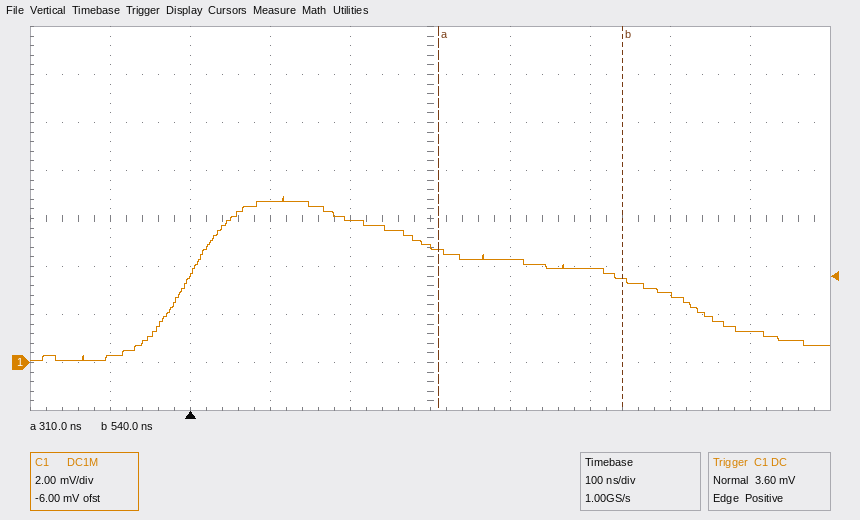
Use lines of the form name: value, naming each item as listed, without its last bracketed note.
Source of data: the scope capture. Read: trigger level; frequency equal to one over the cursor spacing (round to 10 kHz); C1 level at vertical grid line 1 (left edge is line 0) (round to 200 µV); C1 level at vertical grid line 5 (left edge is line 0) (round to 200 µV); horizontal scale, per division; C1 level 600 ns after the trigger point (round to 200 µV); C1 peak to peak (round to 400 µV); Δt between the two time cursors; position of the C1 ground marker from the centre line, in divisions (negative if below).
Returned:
trigger level: 3.60 mV
frequency equal to one over the cursor spacing: 4.35 MHz
C1 level at vertical grid line 1 (left edge is line 0): 200 µV
C1 level at vertical grid line 5 (left edge is line 0): 4.8 mV
horizontal scale, per division: 100 ns
C1 level 600 ns after the trigger point: 2.8 mV
C1 peak to peak: 6.8 mV
Δt between the two time cursors: 230 ns
position of the C1 ground marker from the centre line, in divisions: -3.0 div
